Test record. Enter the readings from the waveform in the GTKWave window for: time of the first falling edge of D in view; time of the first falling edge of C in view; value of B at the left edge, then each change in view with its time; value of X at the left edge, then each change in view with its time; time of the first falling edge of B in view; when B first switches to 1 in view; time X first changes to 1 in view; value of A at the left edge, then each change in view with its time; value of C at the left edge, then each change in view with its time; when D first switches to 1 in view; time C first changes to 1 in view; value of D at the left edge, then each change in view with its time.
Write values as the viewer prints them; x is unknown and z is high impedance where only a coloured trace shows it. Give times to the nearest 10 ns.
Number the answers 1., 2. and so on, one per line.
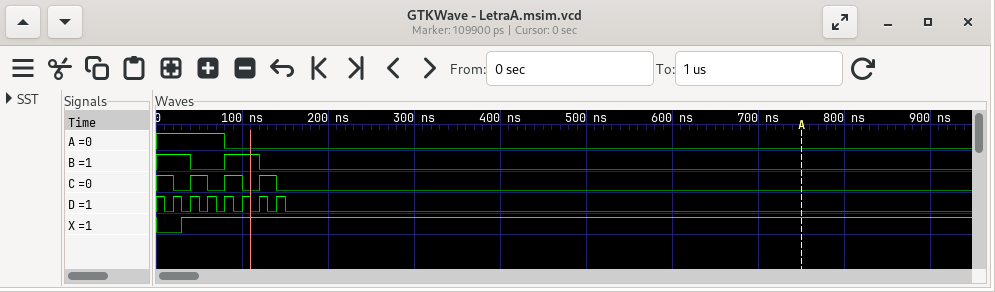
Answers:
1. 10 ns
2. 20 ns
3. 1, 0 at 40 ns, 1 at 80 ns, 0 at 120 ns
4. 0, 1 at 30 ns
5. 40 ns
6. 80 ns
7. 30 ns
8. 1, 0 at 80 ns
9. 1, 0 at 20 ns, 1 at 40 ns, 0 at 60 ns, 1 at 80 ns, 0 at 100 ns, 1 at 120 ns, 0 at 140 ns
10. 20 ns
11. 40 ns
12. 1, 0 at 10 ns, 1 at 20 ns, 0 at 30 ns, 1 at 40 ns, 0 at 50 ns, 1 at 60 ns, 0 at 70 ns, 1 at 80 ns, 0 at 90 ns, 1 at 100 ns, 0 at 110 ns, 1 at 120 ns, 0 at 130 ns, 1 at 140 ns, 0 at 150 ns
